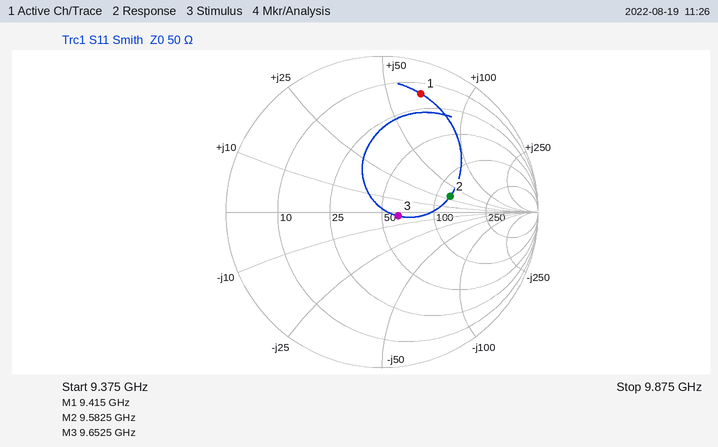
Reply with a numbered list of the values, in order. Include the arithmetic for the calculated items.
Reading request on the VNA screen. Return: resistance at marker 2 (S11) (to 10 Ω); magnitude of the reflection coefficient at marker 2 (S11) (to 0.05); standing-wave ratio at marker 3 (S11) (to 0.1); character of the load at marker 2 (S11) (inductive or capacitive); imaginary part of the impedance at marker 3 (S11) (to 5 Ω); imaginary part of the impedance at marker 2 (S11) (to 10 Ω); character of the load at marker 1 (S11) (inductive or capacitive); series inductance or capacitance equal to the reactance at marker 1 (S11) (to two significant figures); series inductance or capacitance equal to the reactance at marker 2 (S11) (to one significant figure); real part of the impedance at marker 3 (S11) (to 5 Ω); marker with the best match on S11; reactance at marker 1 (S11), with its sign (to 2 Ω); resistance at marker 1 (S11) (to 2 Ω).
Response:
1. 120 Ω
2. 0.45
3. 1.2
4. inductive
5. -5 Ω
6. +30 Ω
7. inductive
8. L = 66 Ω/(2π × 9.415 GHz) ≈ 1.1 nH
9. L = 30 Ω/(2π × 9.5825 GHz) ≈ 498 pH, so 500 pH to one significant figure
10. 60 Ω
11. marker 3
12. +66 Ω
13. 16 Ω
